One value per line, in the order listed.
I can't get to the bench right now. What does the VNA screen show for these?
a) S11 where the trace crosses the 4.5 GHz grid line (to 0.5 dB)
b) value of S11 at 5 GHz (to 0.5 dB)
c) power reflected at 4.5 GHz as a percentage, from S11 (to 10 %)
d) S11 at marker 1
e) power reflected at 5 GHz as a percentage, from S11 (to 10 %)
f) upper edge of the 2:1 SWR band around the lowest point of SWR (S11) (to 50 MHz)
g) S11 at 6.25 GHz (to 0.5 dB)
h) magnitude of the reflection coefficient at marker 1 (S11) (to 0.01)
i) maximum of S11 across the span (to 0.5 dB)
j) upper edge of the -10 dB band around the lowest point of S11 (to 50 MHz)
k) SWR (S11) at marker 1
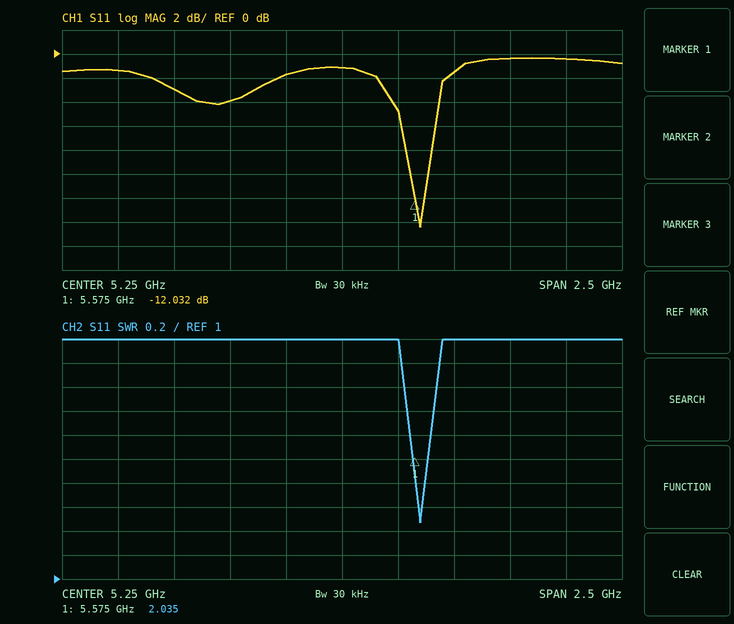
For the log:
-3.0 dB
-1.5 dB
50 %
-12.032 dB
70 %
5.65 GHz
-0.5 dB
0.25
-0.5 dB
5.65 GHz
2.035
